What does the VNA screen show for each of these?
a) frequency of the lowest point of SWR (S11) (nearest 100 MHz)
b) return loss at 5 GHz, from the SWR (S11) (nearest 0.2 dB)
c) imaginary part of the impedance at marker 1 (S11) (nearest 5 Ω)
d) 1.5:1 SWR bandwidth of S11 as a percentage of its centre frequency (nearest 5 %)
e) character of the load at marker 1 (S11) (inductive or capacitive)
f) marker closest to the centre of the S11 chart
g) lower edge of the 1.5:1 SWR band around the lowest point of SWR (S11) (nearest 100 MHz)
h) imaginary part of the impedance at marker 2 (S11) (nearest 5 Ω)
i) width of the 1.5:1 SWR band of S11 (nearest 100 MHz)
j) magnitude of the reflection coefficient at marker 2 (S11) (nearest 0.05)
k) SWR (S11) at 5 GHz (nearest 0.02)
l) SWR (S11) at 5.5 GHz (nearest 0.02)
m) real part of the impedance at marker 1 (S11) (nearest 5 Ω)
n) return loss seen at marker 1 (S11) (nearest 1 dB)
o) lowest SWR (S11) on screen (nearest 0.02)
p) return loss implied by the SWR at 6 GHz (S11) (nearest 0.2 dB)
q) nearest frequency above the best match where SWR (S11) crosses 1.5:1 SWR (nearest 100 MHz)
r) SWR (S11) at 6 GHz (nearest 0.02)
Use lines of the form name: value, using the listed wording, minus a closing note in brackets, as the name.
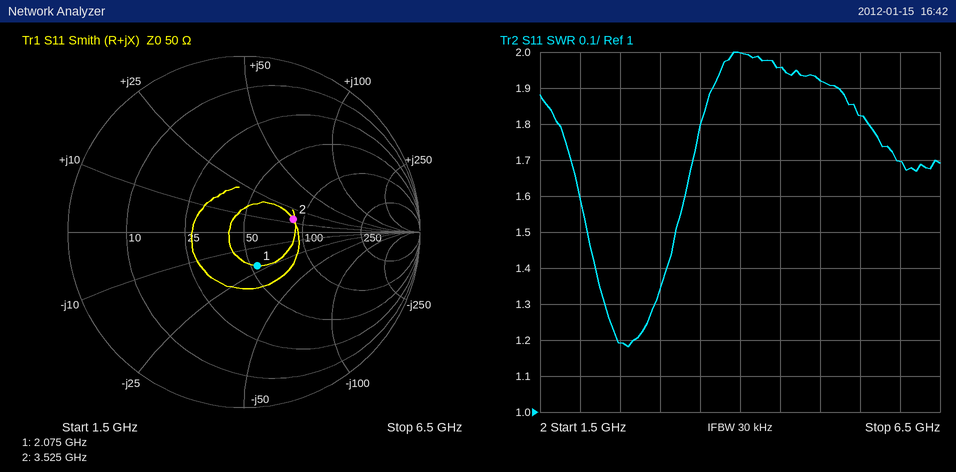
frequency of the lowest point of SWR (S11): 2.6 GHz
return loss at 5 GHz, from the SWR (S11): 10.0 dB
imaginary part of the impedance at marker 1 (S11): -20 Ω
1.5:1 SWR bandwidth of S11 as a percentage of its centre frequency: 40 %
character of the load at marker 1 (S11): capacitive
marker closest to the centre of the S11 chart: marker 1
lower edge of the 1.5:1 SWR band around the lowest point of SWR (S11): 2.1 GHz
imaginary part of the impedance at marker 2 (S11): +15 Ω
width of the 1.5:1 SWR band of S11: 1.1 GHz
magnitude of the reflection coefficient at marker 2 (S11): 0.30
SWR (S11) at 5 GHz: 1.92
SWR (S11) at 5.5 GHz: 1.82
real part of the impedance at marker 1 (S11): 55 Ω
return loss seen at marker 1 (S11): 14 dB
lowest SWR (S11) on screen: 1.18
return loss implied by the SWR at 6 GHz (S11): 11.8 dB
nearest frequency above the best match where SWR (S11) crosses 1.5:1 SWR: 3.2 GHz
SWR (S11) at 6 GHz: 1.70
